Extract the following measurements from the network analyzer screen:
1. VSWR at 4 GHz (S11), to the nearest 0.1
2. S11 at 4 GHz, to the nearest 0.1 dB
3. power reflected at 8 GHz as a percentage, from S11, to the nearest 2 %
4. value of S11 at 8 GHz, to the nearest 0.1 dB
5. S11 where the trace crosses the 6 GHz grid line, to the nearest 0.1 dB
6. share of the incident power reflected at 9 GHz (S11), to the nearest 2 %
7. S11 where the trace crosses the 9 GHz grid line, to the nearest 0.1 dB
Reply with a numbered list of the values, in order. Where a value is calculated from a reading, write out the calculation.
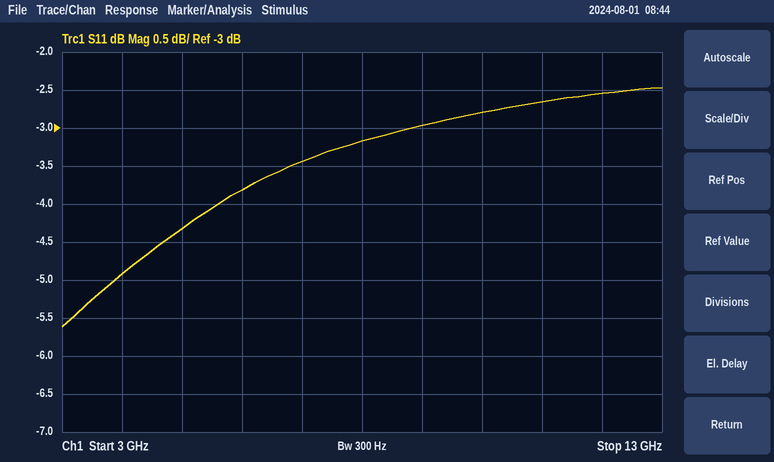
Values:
1. |Γ| = 10^(-4.9/20) = 0.5689; VSWR = (1 + 0.5689)/(1 − 0.5689) ≈ 3.6
2. -4.9 dB
3. 10^(-3.2/10) ≈ 48 %
4. -3.2 dB
5. -3.8 dB
6. 10^(-3/10) ≈ 50 %
7. -3.0 dB
